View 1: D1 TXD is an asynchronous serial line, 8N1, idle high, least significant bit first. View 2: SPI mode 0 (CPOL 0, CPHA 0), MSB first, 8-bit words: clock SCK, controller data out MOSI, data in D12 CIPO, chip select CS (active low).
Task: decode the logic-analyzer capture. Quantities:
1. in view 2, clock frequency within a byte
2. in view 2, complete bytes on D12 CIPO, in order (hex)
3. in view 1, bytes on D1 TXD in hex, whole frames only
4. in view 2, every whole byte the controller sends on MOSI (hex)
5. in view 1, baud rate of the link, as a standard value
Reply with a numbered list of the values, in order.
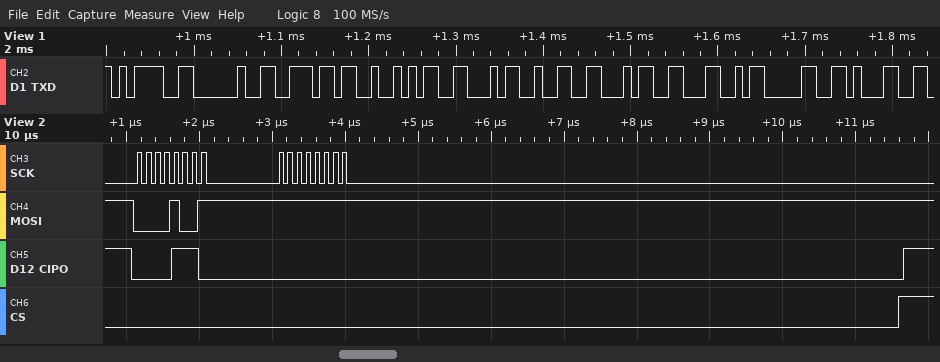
1. 8 MHz
2. 0x0E 0x00
3. 3D 20 6E 52 46 32 34 4C 30 31
4. 0x09 0xFF
5. 115200 baud
